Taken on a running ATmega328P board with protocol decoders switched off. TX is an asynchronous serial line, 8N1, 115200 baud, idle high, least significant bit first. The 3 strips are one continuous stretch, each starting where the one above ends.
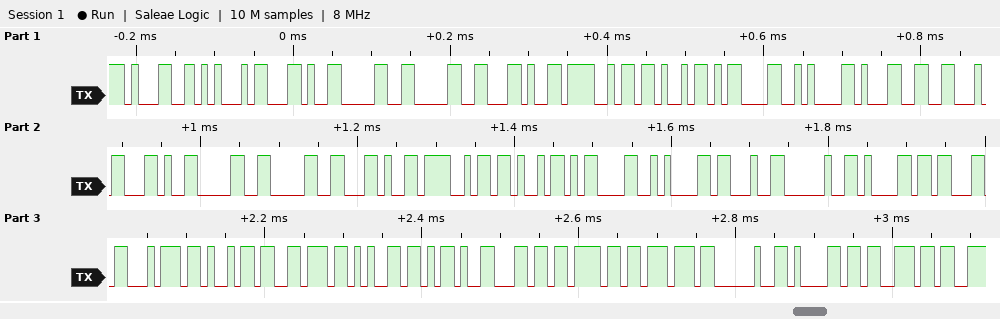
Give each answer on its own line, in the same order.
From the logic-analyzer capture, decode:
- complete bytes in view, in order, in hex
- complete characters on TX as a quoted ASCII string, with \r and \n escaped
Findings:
31 45 2C 30 30 2C 4F 4B 0D 0A 31 46 2C 30 30 2C 4F 4B 0D 0A 23 20 61 63 74 69 76 65 2D 6C 6F 77 20 61 73
"1E,00,OK\r\n1F,00,OK\r\n# active-low as"
